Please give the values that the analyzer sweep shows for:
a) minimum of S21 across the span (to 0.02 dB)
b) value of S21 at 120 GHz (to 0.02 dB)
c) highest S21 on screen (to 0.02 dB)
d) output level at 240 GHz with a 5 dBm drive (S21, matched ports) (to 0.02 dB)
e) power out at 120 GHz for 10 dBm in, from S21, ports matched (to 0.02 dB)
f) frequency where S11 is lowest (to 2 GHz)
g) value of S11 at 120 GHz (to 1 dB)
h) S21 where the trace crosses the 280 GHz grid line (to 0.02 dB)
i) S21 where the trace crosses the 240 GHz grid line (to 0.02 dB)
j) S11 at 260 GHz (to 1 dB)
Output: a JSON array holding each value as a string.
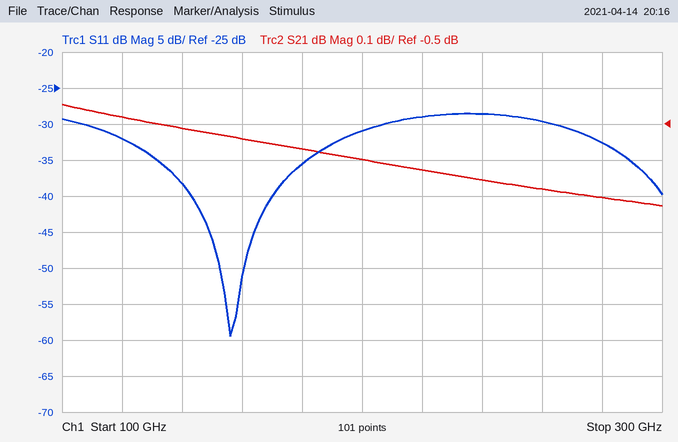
["-0.72 dB", "-0.48 dB", "-0.44 dB", "4.34 dBm", "9.52 dBm", "156 GHz", "-32 dB", "-0.70 dB", "-0.66 dB", "-30 dB"]
